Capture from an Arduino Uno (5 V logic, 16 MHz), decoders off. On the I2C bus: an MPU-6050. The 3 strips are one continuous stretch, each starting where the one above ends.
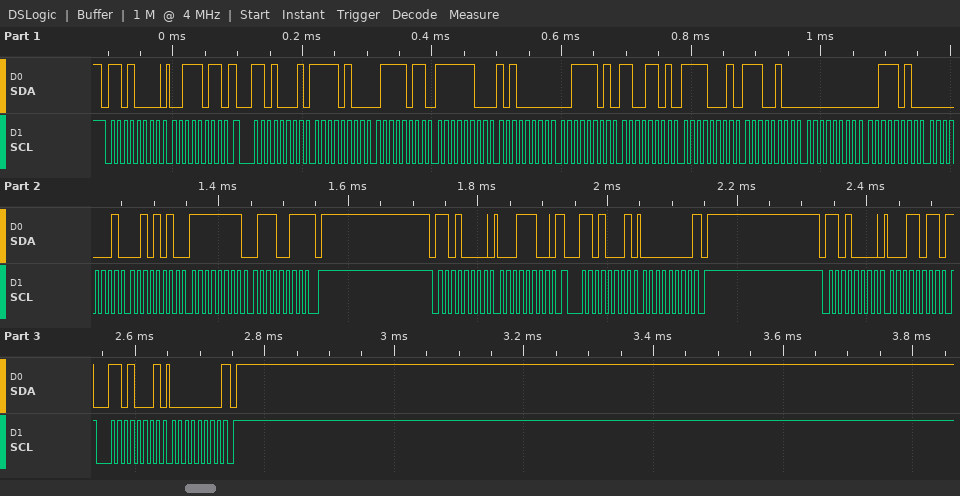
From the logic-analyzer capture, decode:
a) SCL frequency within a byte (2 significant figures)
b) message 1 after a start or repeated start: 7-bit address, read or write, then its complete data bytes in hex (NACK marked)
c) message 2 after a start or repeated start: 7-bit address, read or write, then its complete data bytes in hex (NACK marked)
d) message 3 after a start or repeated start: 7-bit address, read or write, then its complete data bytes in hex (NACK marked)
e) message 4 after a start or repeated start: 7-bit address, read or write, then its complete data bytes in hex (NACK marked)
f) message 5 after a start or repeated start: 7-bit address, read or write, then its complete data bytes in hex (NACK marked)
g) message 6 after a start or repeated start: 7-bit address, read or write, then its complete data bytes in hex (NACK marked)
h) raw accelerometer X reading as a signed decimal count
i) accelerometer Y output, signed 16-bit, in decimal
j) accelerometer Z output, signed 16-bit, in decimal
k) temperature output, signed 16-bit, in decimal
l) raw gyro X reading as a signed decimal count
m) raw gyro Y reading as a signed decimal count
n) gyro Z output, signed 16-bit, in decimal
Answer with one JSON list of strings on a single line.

["100 kHz", "0x68 write: 3B", "0x68 read: F4 7B FC A0 3D CD F1 E4 00 3A 01 2A FF 73 NACK", "0x68 write: 1C", "0x68 read: 00 NACK", "0x68 write: 1B", "0x68 read: 00 NACK", "-2949", "-864", "15821", "-3612", "58", "298", "-141"]
